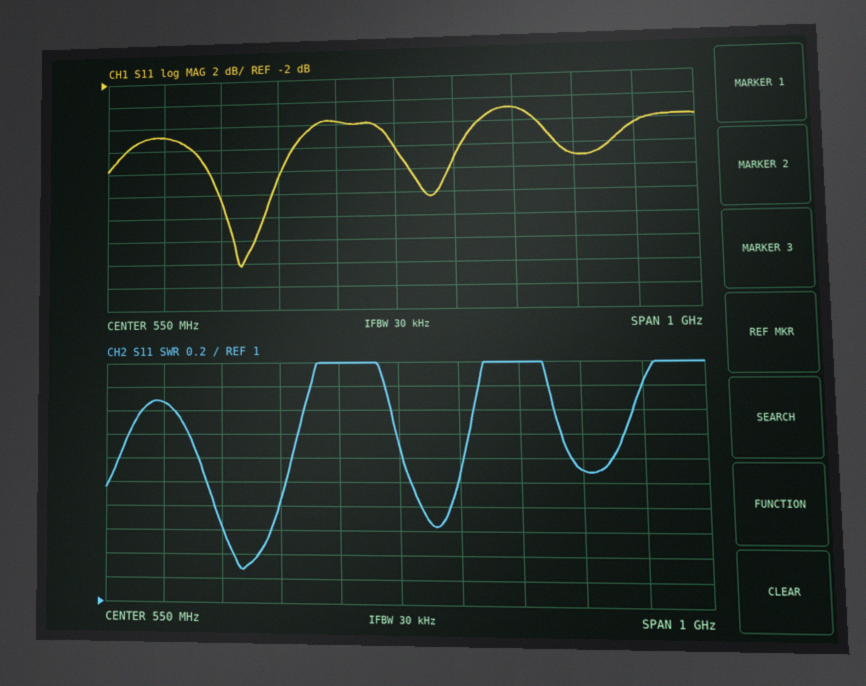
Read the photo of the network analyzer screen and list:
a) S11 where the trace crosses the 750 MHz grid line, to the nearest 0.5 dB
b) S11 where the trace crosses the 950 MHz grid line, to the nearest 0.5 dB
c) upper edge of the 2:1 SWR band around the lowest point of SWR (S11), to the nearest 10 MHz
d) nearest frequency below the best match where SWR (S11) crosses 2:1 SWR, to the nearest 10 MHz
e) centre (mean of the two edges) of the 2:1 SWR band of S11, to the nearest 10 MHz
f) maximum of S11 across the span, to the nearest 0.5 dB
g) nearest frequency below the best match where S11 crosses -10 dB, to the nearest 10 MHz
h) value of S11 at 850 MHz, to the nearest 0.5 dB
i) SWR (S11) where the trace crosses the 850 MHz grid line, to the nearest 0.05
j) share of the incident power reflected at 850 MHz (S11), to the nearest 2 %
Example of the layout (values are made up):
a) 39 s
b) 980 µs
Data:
a) -5.0 dB
b) -6.5 dB
c) 360 MHz
d) 220 MHz
e) 290 MHz
f) -5.0 dB
g) 230 MHz
h) -9.0 dB
i) 2.10
j) 12 %
